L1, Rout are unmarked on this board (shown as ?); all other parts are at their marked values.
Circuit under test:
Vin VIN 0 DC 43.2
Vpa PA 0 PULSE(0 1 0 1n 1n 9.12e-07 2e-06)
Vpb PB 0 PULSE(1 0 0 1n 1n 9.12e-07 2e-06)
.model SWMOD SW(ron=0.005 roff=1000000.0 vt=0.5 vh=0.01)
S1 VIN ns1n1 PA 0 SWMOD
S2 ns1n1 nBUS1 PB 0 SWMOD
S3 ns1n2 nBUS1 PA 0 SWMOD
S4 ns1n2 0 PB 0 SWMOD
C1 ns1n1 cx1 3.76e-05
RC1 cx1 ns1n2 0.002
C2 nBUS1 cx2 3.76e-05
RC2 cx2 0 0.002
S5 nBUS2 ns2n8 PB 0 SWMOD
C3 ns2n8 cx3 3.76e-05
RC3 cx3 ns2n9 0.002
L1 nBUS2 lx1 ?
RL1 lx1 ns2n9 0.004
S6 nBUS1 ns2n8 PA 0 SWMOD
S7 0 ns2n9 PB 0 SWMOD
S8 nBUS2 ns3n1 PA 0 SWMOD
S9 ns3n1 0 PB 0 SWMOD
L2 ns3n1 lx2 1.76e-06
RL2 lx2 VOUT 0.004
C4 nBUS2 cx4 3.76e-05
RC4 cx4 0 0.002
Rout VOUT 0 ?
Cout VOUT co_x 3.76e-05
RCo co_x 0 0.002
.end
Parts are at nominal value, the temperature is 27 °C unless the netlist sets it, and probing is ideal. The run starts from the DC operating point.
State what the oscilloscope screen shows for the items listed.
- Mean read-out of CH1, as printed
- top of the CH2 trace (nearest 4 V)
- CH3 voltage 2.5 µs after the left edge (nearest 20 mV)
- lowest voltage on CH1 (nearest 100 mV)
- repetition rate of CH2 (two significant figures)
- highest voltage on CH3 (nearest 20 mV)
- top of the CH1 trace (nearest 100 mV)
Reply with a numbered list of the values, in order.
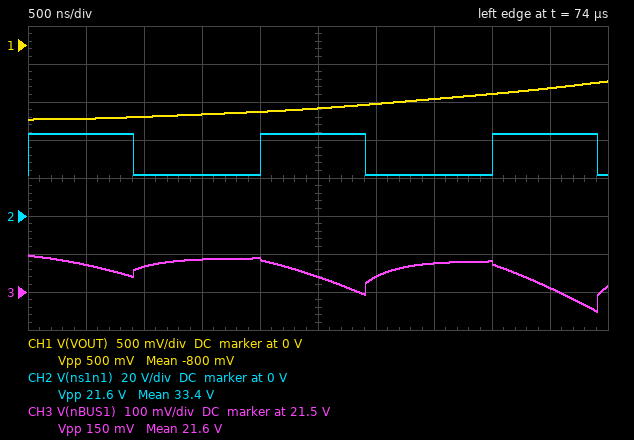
1. -800 mV
2. 44 V
3. 21.54 V
4. -1.0 V
5. 500 kHz
6. 21.60 V
7. -500 mV
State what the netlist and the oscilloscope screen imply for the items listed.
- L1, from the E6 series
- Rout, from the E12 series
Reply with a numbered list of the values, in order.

1. 3.3 µH
2. 1 Ω
